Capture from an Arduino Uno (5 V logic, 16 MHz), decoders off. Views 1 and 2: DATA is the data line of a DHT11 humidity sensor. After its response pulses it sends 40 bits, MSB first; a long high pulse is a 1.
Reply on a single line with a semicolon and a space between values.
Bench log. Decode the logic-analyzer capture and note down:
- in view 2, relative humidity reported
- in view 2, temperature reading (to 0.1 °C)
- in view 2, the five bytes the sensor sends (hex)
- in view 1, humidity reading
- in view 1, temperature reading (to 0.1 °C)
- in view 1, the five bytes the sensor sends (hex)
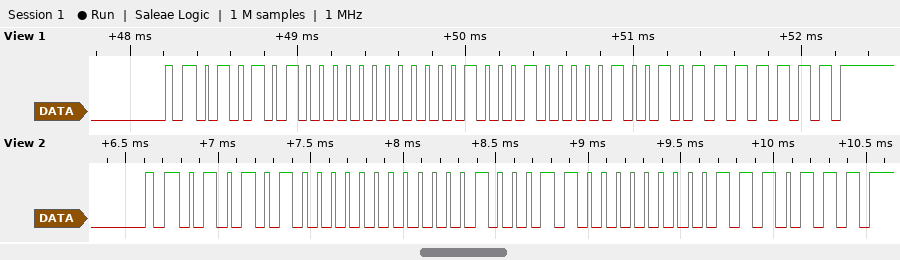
84 %; 35.0 °C; 54 00 23 00 77; 84 %; 34.9 °C; 54 00 22 09 7F
